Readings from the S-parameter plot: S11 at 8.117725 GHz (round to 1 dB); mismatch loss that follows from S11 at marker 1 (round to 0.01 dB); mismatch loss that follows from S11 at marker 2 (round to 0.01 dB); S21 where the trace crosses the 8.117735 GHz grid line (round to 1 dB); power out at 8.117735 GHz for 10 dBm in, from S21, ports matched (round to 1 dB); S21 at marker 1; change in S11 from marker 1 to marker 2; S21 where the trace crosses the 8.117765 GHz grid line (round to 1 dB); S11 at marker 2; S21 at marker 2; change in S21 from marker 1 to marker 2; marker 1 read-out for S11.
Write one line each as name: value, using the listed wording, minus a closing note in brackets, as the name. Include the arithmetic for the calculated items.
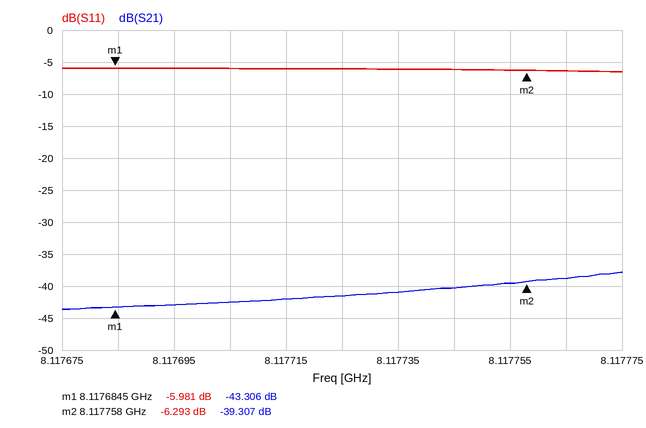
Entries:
S11 at 8.117725 GHz: -6 dB
mismatch loss that follows from S11 at marker 1: −10 log10(1 − 10^(-5.981/10)) ≈ 1.26 dB
mismatch loss that follows from S11 at marker 2: −10 log10(1 − 10^(-6.293/10)) ≈ 1.16 dB
S21 where the trace crosses the 8.117735 GHz grid line: -41 dB
power out at 8.117735 GHz for 10 dBm in, from S21, ports matched: 10 dBm + (-41 dB) = -31 dBm
S21 at marker 1: -43.306 dB
change in S11 from marker 1 to marker 2: -6.293 − (-5.981) = -0.312 dB
S21 where the trace crosses the 8.117765 GHz grid line: -39 dB
S11 at marker 2: -6.293 dB
S21 at marker 2: -39.307 dB
change in S21 from marker 1 to marker 2: -39.307 − (-43.306) = 3.999 dB
marker 1 read-out for S11: -5.981 dB
